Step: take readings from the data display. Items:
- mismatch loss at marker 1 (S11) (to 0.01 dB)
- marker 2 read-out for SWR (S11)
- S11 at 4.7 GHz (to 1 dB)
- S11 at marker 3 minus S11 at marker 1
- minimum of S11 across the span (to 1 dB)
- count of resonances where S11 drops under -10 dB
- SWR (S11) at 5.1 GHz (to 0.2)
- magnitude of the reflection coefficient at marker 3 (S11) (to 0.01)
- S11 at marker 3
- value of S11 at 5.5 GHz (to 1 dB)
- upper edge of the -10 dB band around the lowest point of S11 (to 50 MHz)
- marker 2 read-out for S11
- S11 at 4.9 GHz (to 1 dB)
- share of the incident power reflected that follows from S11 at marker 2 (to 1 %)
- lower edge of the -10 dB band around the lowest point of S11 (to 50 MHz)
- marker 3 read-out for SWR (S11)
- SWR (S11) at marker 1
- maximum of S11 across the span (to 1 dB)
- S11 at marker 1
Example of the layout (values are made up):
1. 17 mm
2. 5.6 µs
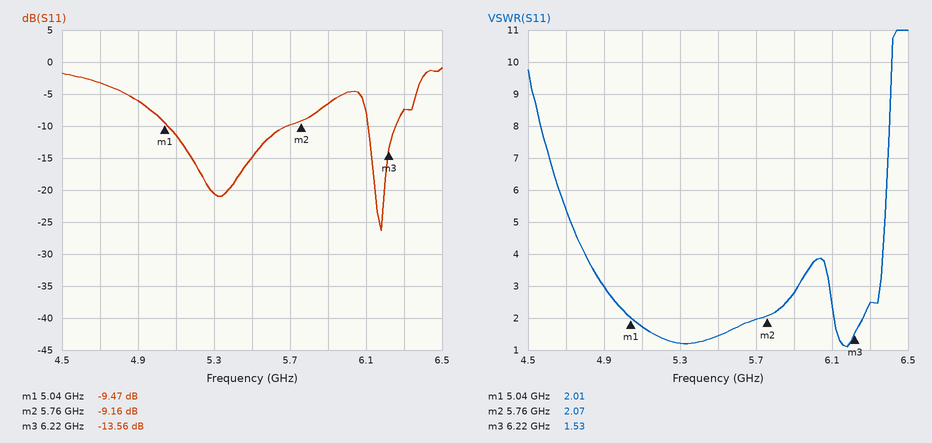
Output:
1. 0.52 dB
2. 2.07
3. -3 dB
4. -4.09 dB
5. -26 dB
6. 2
7. 1.8
8. 0.21
9. -13.56 dB
10. -15 dB
11. 6.25 GHz
12. -9.16 dB
13. -6 dB
14. 12 %
15. 6.10 GHz
16. 1.53
17. 2.01
18. -1 dB
19. -9.47 dB
